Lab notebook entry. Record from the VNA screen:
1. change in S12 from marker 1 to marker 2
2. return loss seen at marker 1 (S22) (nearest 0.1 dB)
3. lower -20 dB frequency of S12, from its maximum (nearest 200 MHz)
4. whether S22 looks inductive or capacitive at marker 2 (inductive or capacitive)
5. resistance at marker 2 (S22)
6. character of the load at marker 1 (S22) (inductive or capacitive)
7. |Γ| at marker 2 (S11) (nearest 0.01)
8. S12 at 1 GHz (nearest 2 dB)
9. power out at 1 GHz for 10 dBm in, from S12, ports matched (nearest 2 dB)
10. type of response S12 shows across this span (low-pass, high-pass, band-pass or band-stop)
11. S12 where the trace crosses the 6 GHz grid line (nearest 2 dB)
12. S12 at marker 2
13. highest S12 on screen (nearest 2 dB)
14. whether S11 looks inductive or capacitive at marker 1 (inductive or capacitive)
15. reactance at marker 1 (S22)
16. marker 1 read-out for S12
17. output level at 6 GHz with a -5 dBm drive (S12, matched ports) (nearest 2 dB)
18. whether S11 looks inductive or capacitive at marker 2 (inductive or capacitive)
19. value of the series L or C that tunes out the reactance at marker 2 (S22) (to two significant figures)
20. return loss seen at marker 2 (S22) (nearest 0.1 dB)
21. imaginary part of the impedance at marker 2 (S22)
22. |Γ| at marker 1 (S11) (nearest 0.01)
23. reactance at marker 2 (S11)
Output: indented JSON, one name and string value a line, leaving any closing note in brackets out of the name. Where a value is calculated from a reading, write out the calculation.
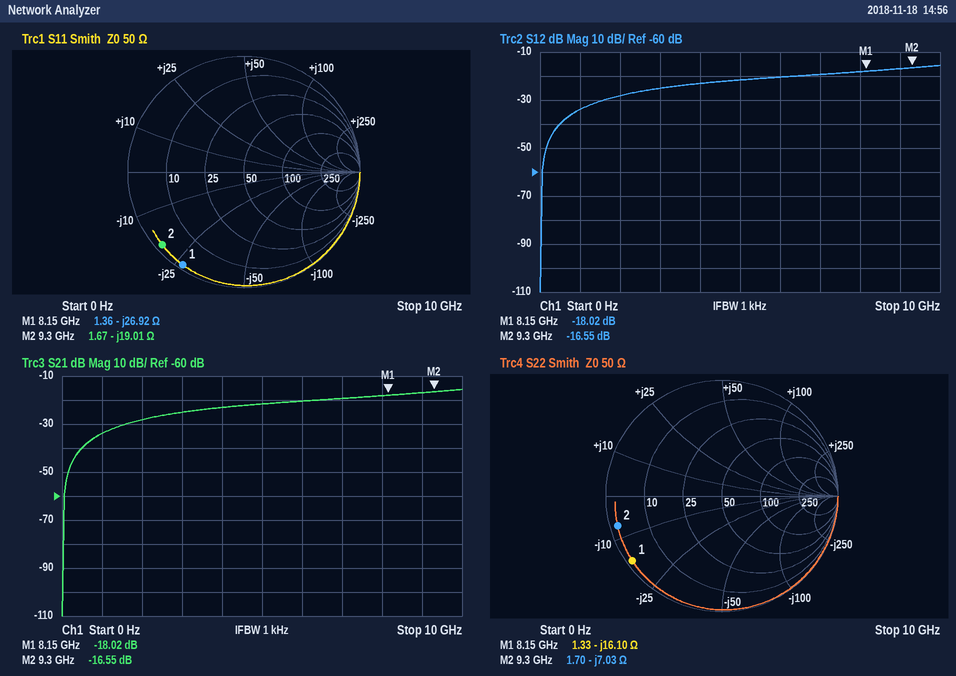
{
  "change in S12 from marker 1 to marker 2": "-16.55 − (-18.02) = 1.47 dB",
  "return loss seen at marker 1 (S22)": "0.4 dB",
  "lower -20 dB frequency of S12, from its maximum": "800 MHz",
  "whether S22 looks inductive or capacitive at marker 2": "capacitive",
  "resistance at marker 2": "1.70 Ω",
  "character of the load at marker 1 (S22)": "capacitive",
  "|Γ| at marker 2 (S11)": "0.94",
  "S12 at 1 GHz": "-34 dB",
  "power out at 1 GHz for 10 dBm in, from S12, ports matched": "10 dBm + (-34 dB) = -24 dBm",
  "type of response S12 shows across this span": "high-pass",
  "S12 where the trace crosses the 6 GHz grid line": "-20 dB",
  "S12 at marker 2": "-16.55 dB",
  "highest S12 on screen": "-16 dB",
  "whether S11 looks inductive or capacitive at marker 1": "capacitive",
  "reactance at marker 1": "-16.10 Ω",
  "marker 1 read-out for S12": "-18.02 dB",
  "output level at 6 GHz with a -5 dBm drive (S12, matched ports)": "-5 dBm + (-20 dB) = -26 dBm",
  "whether S11 looks inductive or capacitive at marker 2": "capacitive",
  "value of the series L or C that tunes out the reactance at marker 2 (S22)": "L = 7.03 Ω/(2π × 9.3 GHz) ≈ 120 pH",
  "return loss seen at marker 2 (S22)": "0.6 dB",
  "imaginary part of the impedance at marker 2": "-7.03 Ω",
  "|Γ| at marker 1 (S11)": "0.96",
  "reactance at marker 2": "-19.01 Ω"
}
